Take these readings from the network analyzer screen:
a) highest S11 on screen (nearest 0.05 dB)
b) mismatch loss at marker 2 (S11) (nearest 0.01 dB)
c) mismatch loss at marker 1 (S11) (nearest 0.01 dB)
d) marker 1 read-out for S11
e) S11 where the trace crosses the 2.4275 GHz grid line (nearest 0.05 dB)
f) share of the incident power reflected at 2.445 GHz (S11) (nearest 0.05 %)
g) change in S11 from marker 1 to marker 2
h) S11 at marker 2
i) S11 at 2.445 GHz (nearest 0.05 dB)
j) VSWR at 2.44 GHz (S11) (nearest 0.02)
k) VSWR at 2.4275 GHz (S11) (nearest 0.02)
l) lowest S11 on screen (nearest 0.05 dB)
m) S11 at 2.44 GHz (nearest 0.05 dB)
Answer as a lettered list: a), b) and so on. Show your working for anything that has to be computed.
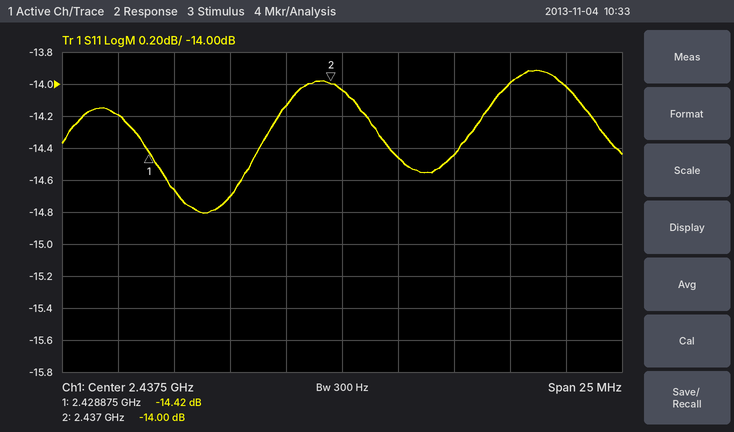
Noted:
a) -13.90 dB
b) −10 log10(1 − 10^(-14/10)) ≈ 0.18 dB
c) −10 log10(1 − 10^(-14.42/10)) ≈ 0.16 dB
d) -14.42 dB
e) -14.20 dB
f) 10^(-14/10) ≈ 3.98 %, so 4.00 % to the nearest 0.05 %
g) -14 − (-14.42) = 0.42 dB
h) -14.00 dB
i) -14.00 dB
j) |Γ| = 10^(-14.45/20) = 0.1895; VSWR = (1 + 0.1895)/(1 − 0.1895) ≈ 1.47, so 1.46 to the nearest 0.02
k) |Γ| = 10^(-14.2/20) = 0.1950; VSWR = (1 + 0.1950)/(1 − 0.1950) ≈ 1.48
l) -14.80 dB
m) -14.45 dB
